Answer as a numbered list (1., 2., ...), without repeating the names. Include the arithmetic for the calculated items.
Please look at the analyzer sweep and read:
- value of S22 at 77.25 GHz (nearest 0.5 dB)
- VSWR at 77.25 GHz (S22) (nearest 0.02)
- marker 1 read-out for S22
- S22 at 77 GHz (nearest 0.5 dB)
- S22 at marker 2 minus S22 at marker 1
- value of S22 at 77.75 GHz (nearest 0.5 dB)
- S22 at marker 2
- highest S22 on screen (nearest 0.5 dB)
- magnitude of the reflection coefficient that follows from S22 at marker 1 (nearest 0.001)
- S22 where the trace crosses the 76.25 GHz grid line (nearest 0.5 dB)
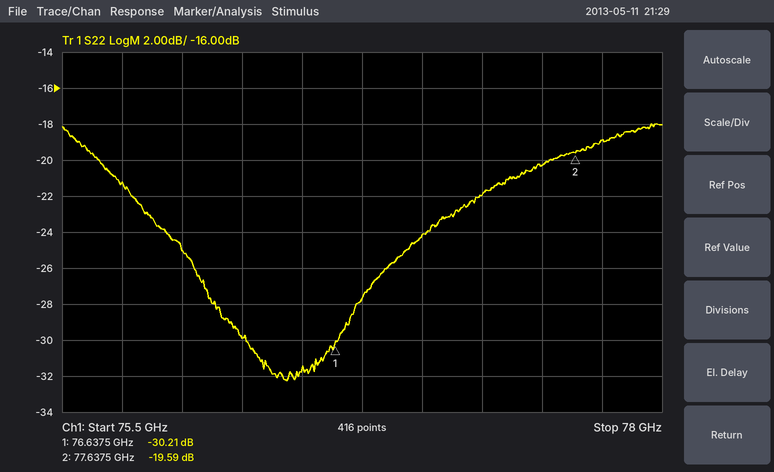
1. -22.0 dB
2. |Γ| = 10^(-22/20) = 0.0794; VSWR = (1 + 0.0794)/(1 − 0.0794) ≈ 1.17, so 1.18 to the nearest 0.02
3. -30.21 dB
4. -24.0 dB
5. -19.59 − (-30.21) = 10.62 dB
6. -19.0 dB
7. -19.59 dB
8. -18.0 dB
9. 10^(-30.21/20) ≈ 0.031
10. -30.0 dB
